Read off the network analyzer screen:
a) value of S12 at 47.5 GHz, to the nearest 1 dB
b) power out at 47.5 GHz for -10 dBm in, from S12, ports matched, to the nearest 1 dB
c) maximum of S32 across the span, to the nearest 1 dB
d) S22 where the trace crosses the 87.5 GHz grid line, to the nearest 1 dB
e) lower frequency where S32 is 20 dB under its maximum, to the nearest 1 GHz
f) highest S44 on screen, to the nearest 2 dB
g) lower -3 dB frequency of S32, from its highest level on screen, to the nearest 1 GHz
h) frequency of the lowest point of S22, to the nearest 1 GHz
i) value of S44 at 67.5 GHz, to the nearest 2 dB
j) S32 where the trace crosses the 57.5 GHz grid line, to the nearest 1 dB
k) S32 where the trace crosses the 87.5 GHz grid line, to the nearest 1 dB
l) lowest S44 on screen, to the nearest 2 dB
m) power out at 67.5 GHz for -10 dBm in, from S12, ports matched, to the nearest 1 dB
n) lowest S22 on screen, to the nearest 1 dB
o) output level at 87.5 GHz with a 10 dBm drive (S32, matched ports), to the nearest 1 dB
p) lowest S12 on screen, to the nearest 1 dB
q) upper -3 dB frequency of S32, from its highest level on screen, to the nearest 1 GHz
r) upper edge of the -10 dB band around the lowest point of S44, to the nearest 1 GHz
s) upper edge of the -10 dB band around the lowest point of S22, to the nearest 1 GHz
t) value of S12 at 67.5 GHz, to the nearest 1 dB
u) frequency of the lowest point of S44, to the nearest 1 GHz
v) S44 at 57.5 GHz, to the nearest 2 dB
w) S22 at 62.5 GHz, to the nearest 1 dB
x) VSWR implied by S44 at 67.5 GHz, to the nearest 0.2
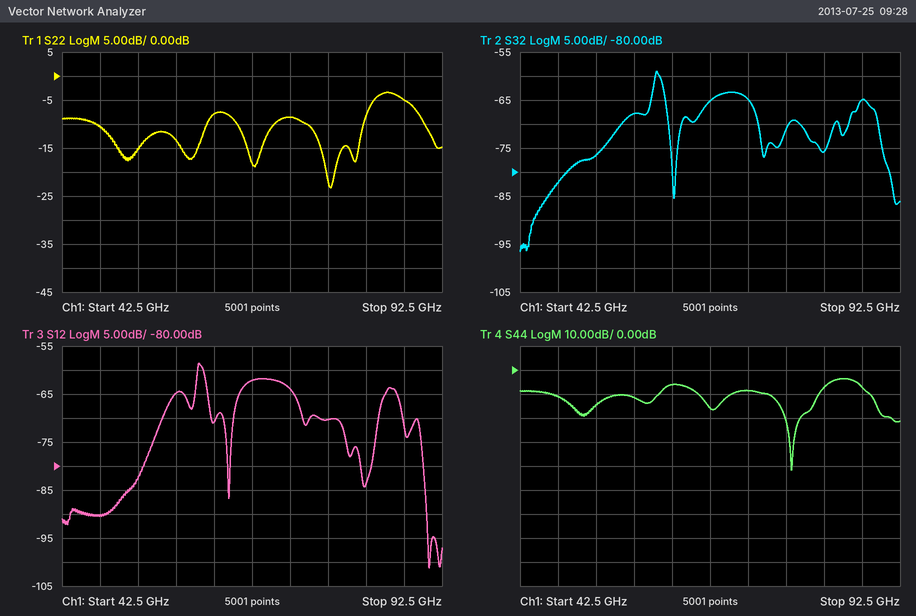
-90 dB
-100 dBm
-59 dB
-5 dB
49 GHz
-4 dB
60 GHz
78 GHz
-16 dB
-68 dB
-65 dB
-42 dB
-72 dBm
-23 dB
-55 dBm
-101 dB
61 GHz
82 GHz
82 GHz
-62 dB
78 GHz
-12 dB
-8 dB
1.4
